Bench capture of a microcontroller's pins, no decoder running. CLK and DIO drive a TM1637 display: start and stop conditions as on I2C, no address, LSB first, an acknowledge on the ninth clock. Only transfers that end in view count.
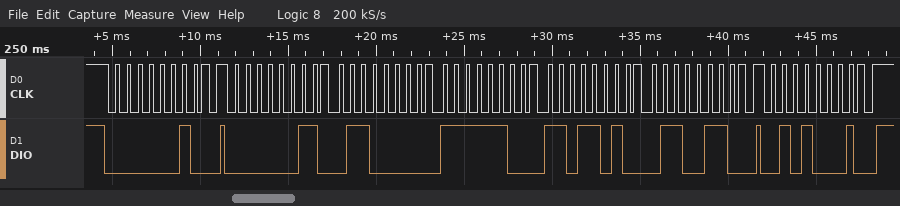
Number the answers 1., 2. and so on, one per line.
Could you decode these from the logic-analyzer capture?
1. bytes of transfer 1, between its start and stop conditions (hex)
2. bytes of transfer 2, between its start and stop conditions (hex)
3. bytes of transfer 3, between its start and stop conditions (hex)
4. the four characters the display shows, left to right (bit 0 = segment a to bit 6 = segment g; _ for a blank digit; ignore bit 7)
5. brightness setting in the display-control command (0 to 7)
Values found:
1. 40
2. C0 06 3F 5B 66
3. 8A
4. 1024
5. 2
